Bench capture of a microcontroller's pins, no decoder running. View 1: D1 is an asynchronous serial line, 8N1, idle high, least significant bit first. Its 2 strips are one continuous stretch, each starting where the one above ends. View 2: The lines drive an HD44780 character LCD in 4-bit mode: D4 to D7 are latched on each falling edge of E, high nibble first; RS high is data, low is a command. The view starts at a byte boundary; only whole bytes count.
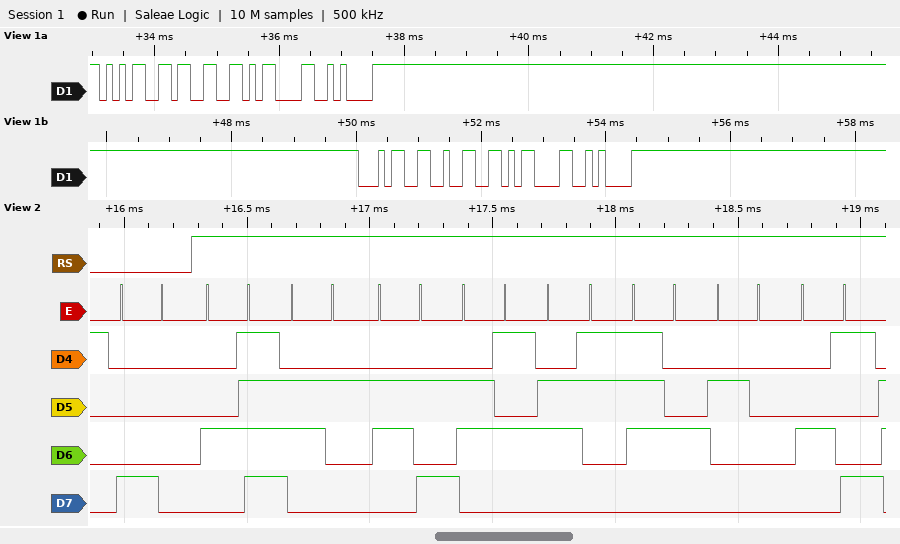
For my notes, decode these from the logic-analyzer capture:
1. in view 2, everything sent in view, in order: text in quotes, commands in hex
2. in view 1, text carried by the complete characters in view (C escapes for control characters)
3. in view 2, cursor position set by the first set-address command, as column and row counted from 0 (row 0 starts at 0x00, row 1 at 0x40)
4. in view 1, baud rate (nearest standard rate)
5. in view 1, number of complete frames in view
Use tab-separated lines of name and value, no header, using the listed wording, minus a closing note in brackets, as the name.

in view 2, everything sent in view, in order: text in quotes, commands in hex	0x80 "Object I"
in view 1, text carried by the complete characters in view	"53\r\n42\r\n"
in view 2, cursor position set by the first set-address command, as column and row counted from 0	column 0, row 0
in view 1, baud rate	9600 baud
in view 1, number of complete frames in view	8
